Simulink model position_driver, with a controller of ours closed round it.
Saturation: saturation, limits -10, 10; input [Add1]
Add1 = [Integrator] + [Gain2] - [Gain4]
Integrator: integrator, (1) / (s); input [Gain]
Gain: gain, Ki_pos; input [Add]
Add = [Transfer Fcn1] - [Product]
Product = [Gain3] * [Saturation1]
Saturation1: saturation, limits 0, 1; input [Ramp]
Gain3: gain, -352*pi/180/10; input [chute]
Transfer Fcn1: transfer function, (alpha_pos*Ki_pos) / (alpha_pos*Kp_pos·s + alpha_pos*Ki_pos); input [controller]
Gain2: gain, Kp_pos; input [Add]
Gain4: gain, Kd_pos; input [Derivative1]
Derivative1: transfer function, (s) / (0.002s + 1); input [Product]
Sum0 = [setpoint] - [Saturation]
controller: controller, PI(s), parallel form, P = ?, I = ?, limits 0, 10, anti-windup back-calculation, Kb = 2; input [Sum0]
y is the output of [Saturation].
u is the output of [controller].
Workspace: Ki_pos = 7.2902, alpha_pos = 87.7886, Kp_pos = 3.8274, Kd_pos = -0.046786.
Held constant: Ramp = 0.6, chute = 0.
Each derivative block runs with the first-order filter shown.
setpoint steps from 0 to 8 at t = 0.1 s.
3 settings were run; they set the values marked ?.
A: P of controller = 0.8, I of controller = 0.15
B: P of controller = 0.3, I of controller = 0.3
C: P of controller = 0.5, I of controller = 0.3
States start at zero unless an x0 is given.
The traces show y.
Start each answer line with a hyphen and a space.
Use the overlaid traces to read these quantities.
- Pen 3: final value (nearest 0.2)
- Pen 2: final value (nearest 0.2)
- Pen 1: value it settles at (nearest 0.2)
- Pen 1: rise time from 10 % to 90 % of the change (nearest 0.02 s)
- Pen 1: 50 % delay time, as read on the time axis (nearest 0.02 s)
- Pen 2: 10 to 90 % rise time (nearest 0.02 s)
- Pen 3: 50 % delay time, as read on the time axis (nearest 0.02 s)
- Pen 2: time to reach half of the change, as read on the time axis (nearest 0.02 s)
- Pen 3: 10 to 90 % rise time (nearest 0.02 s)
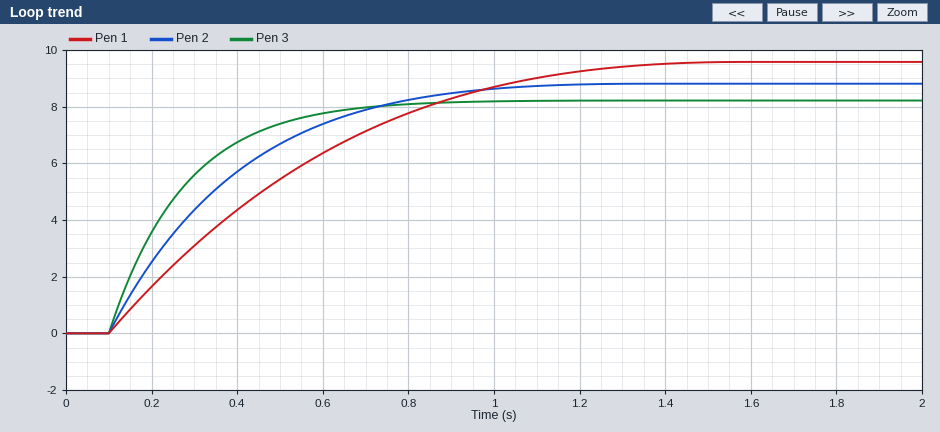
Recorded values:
- 8.2
- 8.8
- 9.6
- 0.82 s
- 0.44 s
- 0.58 s
- 0.22 s
- 0.30 s
- 0.38 s
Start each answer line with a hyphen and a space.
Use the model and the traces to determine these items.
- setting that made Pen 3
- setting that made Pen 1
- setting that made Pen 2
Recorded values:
- A
- B
- C
